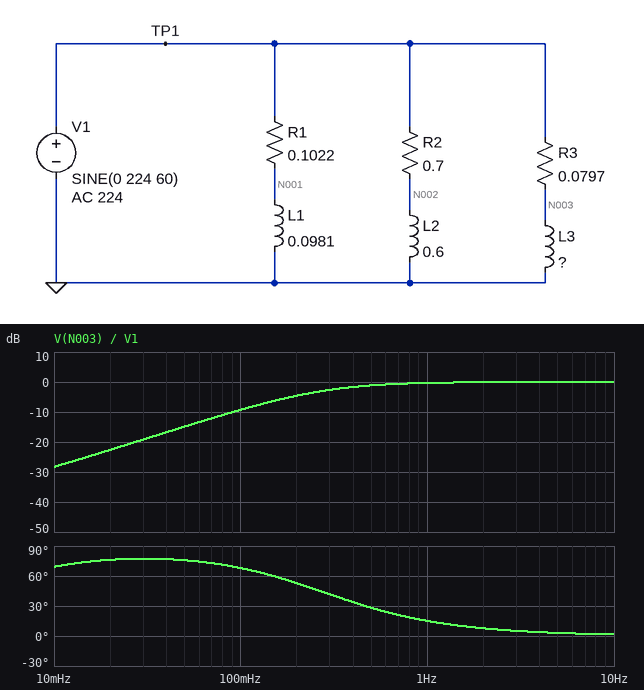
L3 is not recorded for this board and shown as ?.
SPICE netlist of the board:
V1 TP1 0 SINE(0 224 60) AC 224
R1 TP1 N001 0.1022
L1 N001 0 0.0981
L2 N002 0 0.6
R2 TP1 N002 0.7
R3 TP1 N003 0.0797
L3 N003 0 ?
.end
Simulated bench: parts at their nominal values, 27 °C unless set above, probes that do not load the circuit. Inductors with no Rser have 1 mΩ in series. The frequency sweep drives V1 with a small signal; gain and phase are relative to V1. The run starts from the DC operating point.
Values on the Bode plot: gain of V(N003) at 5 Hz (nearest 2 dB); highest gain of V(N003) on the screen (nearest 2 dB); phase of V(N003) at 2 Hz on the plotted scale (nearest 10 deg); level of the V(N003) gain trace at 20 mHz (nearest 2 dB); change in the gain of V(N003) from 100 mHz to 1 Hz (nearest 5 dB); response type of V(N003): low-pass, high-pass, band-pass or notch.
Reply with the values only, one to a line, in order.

0 dB
0 dB
10 deg
-22 dB
10 dB
high-pass
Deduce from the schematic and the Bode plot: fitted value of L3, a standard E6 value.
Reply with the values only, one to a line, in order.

47 mH
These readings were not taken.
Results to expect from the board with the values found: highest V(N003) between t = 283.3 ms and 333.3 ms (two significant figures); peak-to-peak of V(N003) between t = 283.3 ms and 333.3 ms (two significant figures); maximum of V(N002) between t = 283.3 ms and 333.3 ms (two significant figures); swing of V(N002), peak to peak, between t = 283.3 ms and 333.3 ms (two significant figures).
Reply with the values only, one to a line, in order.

220 V
450 V
220 V
450 V
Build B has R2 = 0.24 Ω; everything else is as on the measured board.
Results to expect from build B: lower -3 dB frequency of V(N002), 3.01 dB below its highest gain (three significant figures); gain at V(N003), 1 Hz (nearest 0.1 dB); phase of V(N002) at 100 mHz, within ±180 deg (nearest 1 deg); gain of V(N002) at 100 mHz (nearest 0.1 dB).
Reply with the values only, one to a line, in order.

63.9 mHz
-0.3 dB
32 deg
-1.5 dB
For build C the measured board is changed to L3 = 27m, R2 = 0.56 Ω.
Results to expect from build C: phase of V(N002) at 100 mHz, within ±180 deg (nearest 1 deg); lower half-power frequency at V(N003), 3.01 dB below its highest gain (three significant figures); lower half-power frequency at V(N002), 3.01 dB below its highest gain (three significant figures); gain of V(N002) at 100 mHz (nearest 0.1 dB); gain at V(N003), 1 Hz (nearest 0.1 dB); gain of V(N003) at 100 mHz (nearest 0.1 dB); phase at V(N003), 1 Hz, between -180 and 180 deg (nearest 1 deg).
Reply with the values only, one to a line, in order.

56 deg
476 mHz
149 mHz
-5.1 dB
-0.9 dB
-13.7 dB
25 deg
